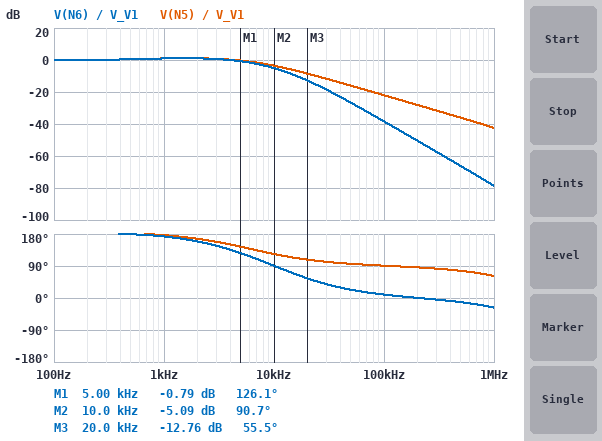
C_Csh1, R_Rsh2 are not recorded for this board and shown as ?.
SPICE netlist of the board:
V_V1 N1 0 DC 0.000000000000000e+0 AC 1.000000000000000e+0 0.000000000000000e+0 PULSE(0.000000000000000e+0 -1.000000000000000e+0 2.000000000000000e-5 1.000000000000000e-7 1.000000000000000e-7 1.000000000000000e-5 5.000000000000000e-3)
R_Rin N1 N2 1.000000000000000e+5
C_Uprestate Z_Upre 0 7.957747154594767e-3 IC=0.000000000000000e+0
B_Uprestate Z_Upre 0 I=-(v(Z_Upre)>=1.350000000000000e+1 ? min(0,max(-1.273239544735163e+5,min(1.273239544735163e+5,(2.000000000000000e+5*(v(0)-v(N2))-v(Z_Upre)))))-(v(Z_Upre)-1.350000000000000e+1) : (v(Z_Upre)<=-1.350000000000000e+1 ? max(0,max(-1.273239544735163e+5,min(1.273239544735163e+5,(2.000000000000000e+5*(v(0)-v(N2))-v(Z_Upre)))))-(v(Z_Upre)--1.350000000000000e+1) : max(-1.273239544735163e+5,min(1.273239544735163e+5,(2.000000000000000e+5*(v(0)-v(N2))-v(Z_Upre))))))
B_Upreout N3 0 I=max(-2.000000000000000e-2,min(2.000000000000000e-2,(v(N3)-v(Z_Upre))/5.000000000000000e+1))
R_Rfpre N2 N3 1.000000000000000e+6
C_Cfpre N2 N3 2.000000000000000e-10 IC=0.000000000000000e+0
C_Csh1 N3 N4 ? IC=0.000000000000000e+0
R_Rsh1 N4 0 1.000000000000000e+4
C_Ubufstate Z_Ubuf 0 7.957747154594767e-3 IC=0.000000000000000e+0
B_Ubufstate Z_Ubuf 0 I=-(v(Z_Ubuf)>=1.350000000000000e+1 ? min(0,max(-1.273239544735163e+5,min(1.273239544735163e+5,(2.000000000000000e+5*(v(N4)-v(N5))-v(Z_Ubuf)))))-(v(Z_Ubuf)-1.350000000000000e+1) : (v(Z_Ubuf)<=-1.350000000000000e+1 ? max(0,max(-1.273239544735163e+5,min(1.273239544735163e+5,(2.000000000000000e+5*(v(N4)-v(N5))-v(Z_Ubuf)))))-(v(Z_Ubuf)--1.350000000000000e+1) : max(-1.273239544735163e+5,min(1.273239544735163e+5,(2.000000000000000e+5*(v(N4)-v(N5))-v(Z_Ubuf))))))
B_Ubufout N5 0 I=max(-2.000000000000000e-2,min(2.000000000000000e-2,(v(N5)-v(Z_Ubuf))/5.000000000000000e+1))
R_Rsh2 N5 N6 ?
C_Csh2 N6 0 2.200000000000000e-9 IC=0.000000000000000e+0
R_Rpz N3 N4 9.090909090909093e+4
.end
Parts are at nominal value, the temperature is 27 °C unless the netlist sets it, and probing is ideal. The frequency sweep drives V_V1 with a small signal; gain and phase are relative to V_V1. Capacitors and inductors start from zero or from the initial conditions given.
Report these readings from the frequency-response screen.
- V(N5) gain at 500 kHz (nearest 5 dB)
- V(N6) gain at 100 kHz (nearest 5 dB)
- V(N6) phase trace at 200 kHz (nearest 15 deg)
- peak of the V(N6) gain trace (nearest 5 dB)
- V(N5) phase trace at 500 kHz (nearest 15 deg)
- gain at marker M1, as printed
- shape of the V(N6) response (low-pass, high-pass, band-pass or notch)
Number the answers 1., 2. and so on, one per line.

1. -35 dB
2. -40 dB
3. 0 deg
4. 0 dB
5. 75 deg
6. -0.79 dB
7. low-pass
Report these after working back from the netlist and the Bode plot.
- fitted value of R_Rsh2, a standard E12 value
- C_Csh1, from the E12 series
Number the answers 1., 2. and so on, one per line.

1. 4.7 kΩ
2. 2.7 nF
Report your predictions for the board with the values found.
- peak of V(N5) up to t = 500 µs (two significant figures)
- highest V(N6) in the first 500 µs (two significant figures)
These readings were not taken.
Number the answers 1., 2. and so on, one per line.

1. 410 mV
2. 260 mV
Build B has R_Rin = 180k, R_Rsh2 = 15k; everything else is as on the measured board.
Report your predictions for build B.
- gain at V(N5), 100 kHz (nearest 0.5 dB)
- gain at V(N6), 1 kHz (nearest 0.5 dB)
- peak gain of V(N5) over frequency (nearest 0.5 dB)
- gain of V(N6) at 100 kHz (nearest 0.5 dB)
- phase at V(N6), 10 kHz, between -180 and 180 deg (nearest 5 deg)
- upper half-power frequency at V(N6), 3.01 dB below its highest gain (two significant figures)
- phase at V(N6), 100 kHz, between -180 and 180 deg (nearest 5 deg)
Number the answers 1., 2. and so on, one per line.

1. -27.0 dB
2. -4.5 dB
3. -4.0 dB
4. -53.5 dB
5. 60 deg
6. 4.1 kHz
7. 5 deg
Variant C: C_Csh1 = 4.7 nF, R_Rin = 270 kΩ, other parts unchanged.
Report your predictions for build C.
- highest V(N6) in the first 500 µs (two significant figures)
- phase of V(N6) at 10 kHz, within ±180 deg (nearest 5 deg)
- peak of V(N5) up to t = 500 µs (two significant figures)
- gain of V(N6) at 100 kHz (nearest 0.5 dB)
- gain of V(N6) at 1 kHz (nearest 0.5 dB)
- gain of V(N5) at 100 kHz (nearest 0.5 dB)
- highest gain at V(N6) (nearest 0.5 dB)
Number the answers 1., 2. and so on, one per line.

1. 110 mV
2. 80 deg
3. 160 mV
4. -47.0 dB
5. -4.0 dB
6. -30.5 dB
7. -3.5 dB
